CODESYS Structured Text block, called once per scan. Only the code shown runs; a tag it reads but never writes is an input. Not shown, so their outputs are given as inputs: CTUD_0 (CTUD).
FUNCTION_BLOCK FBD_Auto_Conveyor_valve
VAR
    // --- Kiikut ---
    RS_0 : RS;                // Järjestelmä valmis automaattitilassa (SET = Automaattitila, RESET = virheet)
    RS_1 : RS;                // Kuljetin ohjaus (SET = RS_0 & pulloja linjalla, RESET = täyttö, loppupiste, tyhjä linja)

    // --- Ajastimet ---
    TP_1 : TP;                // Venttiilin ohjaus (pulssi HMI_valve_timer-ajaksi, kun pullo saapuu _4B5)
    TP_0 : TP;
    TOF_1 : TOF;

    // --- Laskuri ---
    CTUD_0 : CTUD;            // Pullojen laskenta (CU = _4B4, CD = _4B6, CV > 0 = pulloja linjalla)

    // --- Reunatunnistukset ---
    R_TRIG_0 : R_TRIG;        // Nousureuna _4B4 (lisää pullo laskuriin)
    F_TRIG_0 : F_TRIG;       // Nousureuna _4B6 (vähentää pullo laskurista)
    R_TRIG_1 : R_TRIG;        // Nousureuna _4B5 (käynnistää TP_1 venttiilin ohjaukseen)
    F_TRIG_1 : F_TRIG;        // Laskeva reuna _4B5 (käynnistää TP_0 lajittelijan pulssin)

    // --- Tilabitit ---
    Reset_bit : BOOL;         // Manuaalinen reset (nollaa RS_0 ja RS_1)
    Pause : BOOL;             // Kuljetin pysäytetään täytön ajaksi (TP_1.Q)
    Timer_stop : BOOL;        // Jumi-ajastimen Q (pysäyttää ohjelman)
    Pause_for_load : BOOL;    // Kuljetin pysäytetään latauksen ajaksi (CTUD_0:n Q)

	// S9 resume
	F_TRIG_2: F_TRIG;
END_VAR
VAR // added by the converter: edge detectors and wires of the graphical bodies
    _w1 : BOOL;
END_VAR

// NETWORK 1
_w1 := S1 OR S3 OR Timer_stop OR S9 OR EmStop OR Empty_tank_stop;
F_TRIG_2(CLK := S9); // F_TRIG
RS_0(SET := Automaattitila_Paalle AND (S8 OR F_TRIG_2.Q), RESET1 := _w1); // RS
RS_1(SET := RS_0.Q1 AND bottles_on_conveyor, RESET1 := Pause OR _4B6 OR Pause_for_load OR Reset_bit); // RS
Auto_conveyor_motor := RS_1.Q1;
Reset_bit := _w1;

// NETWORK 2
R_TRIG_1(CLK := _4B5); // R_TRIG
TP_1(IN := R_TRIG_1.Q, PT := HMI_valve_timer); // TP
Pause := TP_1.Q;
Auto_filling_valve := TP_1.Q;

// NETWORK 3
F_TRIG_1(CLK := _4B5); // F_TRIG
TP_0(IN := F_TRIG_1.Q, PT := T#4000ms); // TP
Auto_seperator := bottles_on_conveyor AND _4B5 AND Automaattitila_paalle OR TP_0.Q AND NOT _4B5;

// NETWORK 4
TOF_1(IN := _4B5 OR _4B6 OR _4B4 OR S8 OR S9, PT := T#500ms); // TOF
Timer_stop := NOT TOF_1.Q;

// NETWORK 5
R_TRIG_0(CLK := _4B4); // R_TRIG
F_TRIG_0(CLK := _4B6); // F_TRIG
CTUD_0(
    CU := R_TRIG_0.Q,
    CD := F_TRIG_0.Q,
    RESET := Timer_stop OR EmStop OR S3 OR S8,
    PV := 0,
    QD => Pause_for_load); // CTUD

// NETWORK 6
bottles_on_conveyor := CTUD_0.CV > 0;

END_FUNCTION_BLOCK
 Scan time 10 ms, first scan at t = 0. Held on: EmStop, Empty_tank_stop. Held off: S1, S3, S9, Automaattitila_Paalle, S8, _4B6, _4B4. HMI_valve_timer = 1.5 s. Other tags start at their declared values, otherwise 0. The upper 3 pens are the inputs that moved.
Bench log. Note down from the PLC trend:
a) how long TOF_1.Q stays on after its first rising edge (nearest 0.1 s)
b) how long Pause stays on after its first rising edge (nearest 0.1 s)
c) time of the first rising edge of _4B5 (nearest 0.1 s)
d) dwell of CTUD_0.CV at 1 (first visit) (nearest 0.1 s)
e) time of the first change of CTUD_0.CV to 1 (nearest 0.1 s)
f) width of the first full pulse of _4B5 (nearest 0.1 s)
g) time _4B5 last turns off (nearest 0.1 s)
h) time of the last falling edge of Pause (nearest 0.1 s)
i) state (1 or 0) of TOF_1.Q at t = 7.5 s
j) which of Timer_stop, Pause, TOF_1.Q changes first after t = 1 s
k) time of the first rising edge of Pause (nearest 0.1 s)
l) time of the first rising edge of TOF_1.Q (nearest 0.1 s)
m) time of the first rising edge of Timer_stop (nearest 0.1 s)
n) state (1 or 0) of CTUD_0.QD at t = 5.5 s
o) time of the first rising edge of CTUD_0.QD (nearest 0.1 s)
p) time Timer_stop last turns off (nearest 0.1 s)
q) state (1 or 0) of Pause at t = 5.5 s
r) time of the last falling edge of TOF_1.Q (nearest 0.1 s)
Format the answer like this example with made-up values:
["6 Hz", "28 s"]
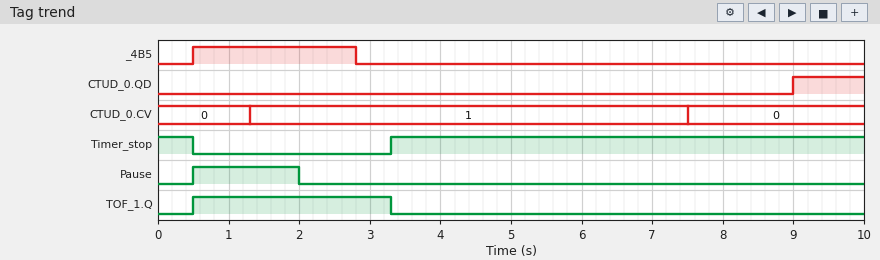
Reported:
["2.8 s", "1.5 s", "0.5 s", "6.2 s", "1.3 s", "2.3 s", "2.8 s", "2.0 s", "0", "Pause", "0.5 s", "0.5 s", "3.3 s", "0", "9.0 s", "0.5 s", "0", "3.3 s"]
